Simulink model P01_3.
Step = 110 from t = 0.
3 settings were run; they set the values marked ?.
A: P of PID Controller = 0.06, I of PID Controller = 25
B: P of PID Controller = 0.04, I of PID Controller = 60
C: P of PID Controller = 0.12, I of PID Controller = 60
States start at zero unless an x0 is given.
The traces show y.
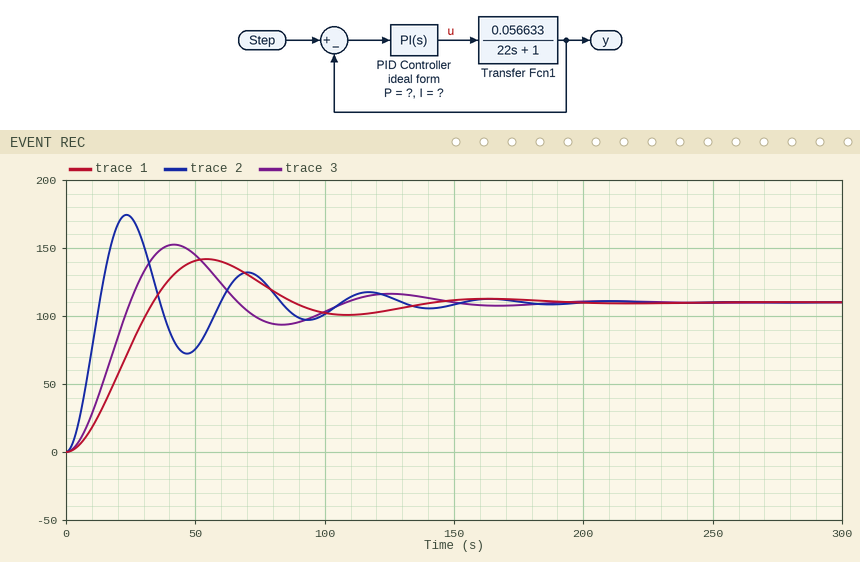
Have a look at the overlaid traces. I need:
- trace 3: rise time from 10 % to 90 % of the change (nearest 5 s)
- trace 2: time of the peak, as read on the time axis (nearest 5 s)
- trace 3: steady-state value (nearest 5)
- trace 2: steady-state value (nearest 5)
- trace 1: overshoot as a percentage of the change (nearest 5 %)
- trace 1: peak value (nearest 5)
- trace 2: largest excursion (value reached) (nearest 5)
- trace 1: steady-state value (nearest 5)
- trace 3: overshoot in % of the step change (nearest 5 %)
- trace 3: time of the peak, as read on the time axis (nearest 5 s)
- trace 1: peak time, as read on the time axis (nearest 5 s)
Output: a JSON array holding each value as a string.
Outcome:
["15 s", "25 s", "110", "110", "30 %", "140", "175", "110", "40 %", "40 s", "55 s"]
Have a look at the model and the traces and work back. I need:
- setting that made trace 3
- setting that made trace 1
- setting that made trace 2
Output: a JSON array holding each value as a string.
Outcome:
["B", "A", "C"]
